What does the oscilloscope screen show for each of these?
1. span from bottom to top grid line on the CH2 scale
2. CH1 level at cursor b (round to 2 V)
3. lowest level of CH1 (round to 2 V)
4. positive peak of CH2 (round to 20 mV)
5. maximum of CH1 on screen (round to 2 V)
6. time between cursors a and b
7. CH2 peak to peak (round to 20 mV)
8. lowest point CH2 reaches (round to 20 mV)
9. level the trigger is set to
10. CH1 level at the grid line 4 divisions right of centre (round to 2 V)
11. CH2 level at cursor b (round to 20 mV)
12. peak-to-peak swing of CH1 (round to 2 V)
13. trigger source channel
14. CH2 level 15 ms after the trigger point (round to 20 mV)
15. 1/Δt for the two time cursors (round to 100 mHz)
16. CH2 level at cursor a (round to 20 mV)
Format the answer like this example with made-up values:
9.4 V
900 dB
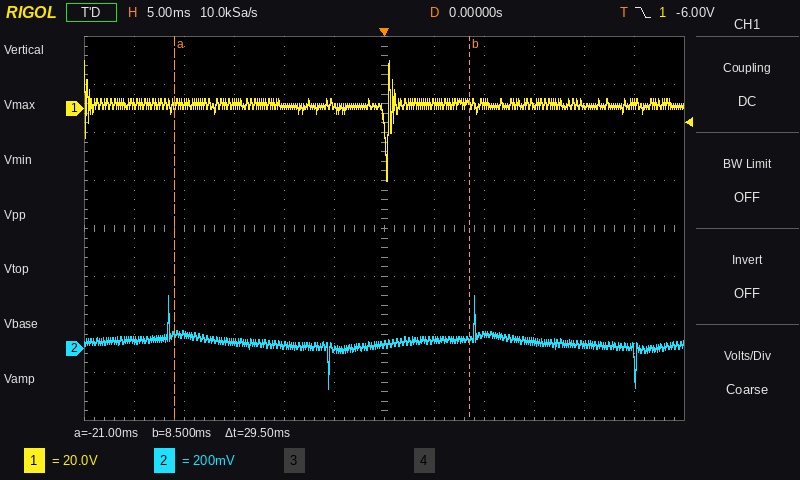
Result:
1.6 V
2 V
-30 V
220 mV
20 V
29.5 ms
380 mV
-160 mV
-6.00 V
2 V
40 mV
50 V
CH1
20 mV
33.9 Hz
60 mV
